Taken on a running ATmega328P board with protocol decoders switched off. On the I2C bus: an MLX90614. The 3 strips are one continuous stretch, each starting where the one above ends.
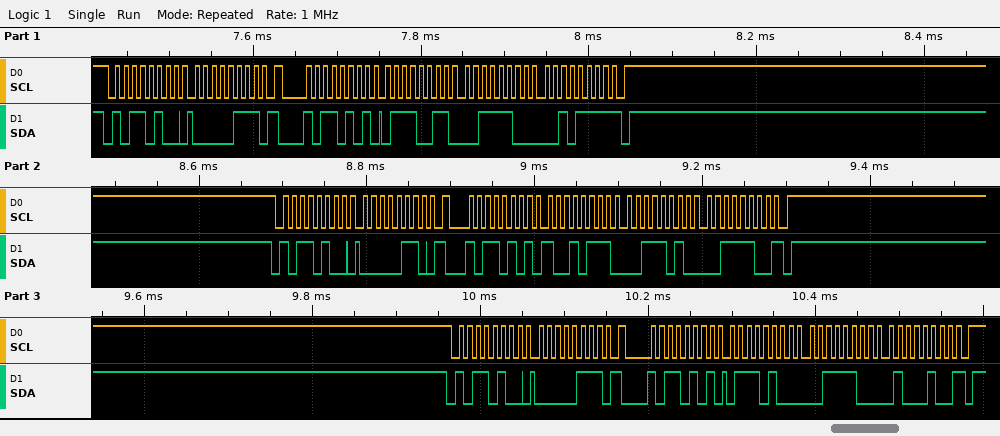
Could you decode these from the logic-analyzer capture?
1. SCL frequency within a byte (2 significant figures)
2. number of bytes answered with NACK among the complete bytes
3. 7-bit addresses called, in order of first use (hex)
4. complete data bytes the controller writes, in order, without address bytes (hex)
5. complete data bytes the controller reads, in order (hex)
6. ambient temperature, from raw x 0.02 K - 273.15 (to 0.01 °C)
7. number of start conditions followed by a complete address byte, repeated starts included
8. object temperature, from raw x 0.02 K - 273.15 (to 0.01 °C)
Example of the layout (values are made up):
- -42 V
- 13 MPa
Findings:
- 100 kHz
- 3
- 0x5A
- 07 06 07
- 73 3C 2F 97 3A 3C 74 3C 44
- 26.83 °C
- 6
- 36.35 °C
